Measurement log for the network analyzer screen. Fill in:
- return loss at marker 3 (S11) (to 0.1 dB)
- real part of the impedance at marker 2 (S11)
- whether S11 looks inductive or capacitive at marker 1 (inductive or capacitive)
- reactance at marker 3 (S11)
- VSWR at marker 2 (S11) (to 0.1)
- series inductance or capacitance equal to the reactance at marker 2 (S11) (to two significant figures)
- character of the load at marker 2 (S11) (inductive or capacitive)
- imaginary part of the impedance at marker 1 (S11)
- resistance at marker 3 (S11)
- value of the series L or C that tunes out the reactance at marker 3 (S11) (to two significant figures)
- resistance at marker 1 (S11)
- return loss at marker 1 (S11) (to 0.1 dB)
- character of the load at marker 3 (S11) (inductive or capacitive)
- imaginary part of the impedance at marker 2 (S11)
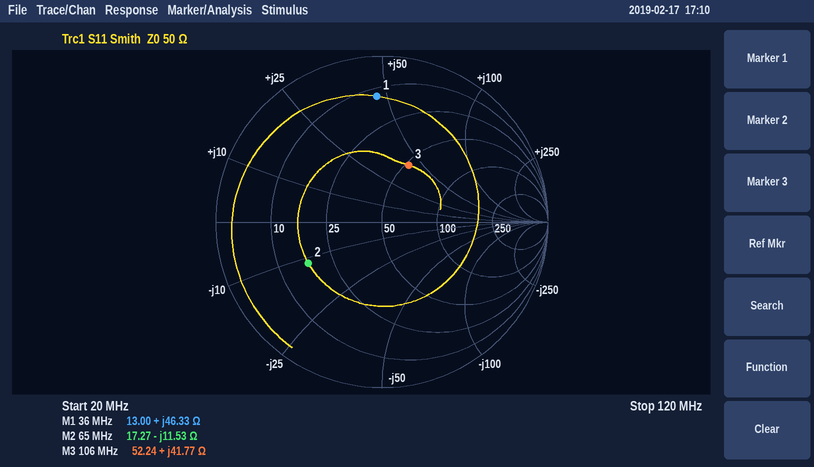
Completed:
8.4 dB
17.27 Ω
inductive
+41.77 Ω
3.1
210 pF
capacitive
+46.33 Ω
52.24 Ω
36 pF
13.00 Ω
2.4 dB
inductive
-11.53 Ω
